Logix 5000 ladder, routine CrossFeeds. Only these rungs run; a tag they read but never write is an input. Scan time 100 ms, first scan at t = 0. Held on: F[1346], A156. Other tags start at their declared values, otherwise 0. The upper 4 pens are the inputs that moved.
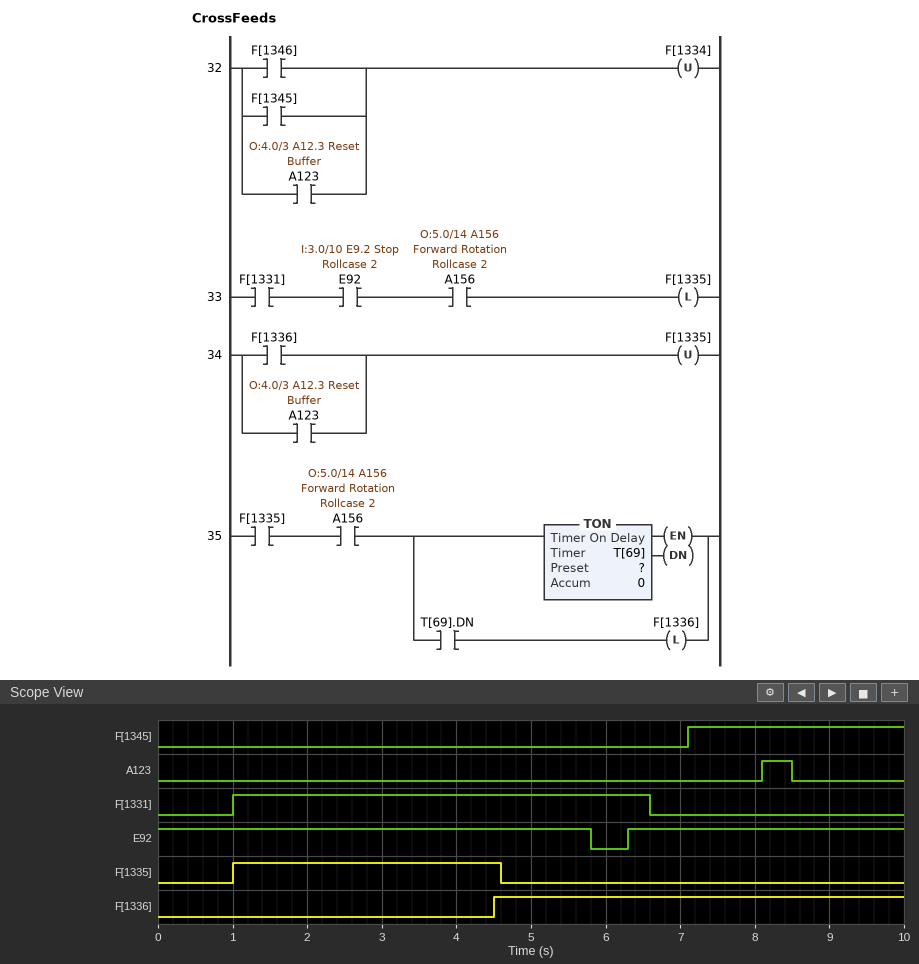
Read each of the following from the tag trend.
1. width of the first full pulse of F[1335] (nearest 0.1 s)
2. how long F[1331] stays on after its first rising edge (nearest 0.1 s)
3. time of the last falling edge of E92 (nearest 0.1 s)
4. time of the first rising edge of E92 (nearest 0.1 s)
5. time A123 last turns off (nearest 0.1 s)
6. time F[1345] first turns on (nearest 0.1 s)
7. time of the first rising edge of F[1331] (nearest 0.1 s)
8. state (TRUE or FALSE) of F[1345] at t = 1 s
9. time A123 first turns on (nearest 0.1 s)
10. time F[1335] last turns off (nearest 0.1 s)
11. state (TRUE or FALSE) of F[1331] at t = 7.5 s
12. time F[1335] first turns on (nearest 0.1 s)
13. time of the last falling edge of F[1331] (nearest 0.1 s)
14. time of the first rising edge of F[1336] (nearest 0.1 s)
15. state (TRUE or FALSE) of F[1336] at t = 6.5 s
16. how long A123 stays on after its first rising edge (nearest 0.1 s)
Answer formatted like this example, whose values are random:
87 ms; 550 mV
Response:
3.6 s; 5.6 s; 5.8 s; 6.3 s; 8.5 s; 7.1 s; 1.0 s; FALSE; 8.1 s; 4.6 s; FALSE; 1.0 s; 6.6 s; 4.5 s; TRUE; 0.4 s
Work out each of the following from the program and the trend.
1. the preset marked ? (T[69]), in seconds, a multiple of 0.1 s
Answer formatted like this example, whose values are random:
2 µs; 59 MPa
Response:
3.5 s
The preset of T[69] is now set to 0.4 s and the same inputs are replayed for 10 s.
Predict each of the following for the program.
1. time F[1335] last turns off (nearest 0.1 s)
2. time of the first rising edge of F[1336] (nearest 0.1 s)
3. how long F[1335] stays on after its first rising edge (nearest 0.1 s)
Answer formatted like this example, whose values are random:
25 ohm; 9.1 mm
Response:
1.5 s; 1.4 s; 0.5 s
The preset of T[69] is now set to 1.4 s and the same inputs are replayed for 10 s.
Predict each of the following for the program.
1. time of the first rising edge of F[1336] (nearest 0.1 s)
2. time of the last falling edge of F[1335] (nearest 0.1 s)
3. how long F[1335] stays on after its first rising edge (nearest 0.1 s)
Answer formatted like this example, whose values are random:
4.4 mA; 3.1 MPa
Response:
2.4 s; 2.5 s; 1.5 s
